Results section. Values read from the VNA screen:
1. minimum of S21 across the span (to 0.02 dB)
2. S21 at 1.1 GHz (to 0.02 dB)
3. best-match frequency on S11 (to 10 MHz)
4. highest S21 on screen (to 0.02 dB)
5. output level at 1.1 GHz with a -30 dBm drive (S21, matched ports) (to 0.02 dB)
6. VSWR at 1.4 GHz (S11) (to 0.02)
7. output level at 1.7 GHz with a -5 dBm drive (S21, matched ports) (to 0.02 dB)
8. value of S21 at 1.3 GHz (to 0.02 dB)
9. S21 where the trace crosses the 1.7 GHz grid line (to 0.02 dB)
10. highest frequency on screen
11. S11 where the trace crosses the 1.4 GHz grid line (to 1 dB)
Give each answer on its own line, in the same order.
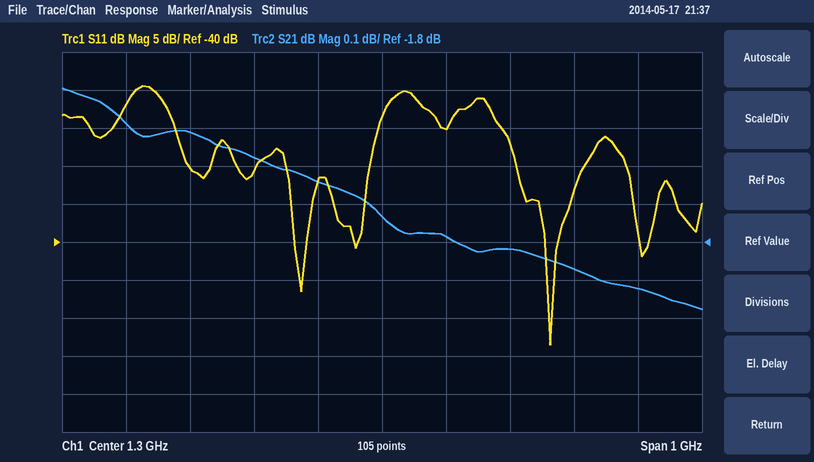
-1.98 dB
-1.58 dB
1.56 GHz
-1.40 dB
-31.58 dBm
1.12
-6.92 dBm
-1.74 dB
-1.92 dB
1.8 GHz
-25 dB
